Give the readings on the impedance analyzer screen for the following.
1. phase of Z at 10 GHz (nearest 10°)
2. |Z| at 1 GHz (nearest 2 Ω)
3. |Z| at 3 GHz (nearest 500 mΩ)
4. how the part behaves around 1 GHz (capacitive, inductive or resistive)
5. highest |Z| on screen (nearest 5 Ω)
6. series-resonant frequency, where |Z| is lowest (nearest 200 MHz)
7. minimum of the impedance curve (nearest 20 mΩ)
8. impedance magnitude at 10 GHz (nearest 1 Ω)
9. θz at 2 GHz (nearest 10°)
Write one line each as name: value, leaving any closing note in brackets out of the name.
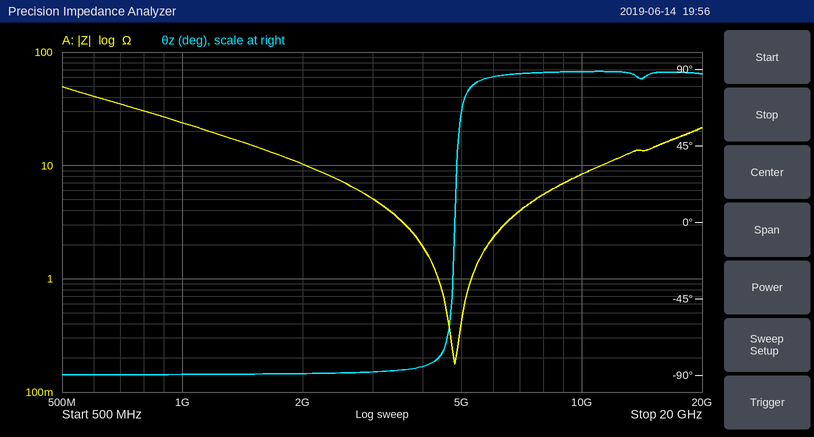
phase of Z at 10 GHz: 90°
|Z| at 1 GHz: 24 Ω
|Z| at 3 GHz: 5.0 Ω
how the part behaves around 1 GHz: capacitive
highest |Z| on screen: 50 Ω
series-resonant frequency, where |Z| is lowest: 4.8 GHz
minimum of the impedance curve: 180 mΩ
impedance magnitude at 10 GHz: 8 Ω
θz at 2 GHz: -90°
